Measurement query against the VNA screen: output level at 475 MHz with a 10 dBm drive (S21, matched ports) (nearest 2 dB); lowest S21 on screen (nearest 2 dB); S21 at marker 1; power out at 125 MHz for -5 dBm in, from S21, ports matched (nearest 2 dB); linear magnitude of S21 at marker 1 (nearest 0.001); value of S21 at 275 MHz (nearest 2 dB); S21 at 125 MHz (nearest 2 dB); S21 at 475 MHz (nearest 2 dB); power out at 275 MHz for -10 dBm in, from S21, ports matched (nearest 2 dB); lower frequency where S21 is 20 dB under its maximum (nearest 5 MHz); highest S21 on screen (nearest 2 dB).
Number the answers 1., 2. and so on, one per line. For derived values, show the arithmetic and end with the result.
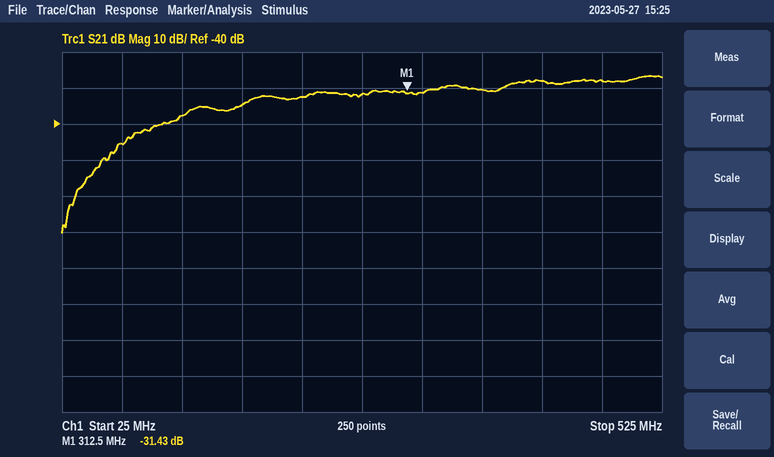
1. 10 dBm + (-28 dB) = -18 dBm
2. -70 dB
3. -31.43 dB
4. -5 dBm + (-38 dB) = -42 dBm
5. 10^(-31.43/20) ≈ 0.027
6. -32 dB
7. -38 dB
8. -28 dB
9. -10 dBm + (-32 dB) = -42 dBm
10. 70 MHz
11. -26 dB
